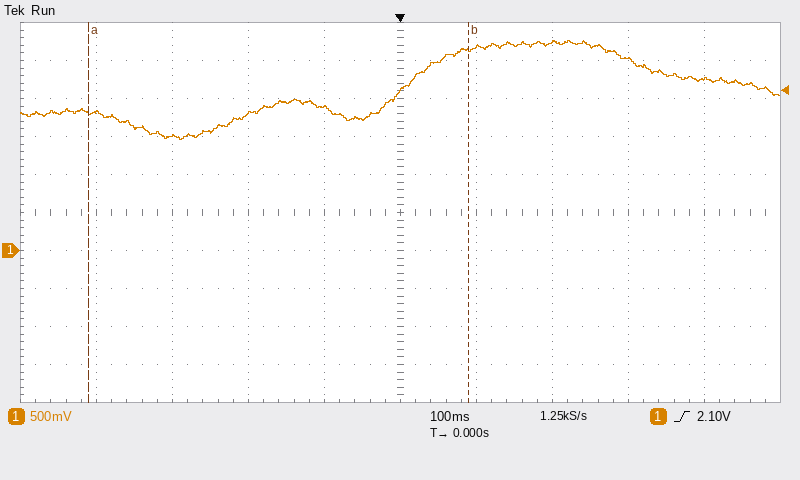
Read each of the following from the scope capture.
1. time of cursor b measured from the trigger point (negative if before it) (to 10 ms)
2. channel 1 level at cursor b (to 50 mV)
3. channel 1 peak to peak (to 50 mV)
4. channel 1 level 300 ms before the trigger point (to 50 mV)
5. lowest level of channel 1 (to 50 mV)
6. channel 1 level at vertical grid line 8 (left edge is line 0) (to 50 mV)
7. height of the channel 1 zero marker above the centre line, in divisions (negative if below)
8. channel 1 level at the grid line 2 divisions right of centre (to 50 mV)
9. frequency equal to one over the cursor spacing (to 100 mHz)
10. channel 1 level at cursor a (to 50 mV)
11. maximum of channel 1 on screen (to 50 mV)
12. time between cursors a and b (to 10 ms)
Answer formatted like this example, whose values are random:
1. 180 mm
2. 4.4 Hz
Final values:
1. +90 ms
2. 2.65 V
3. 1.30 V
4. 1.50 V
5. 1.45 V
6. 2.50 V
7. -1.0 div
8. 2.75 V
9. 2.0 Hz
10. 1.80 V
11. 2.75 V
12. 500 ms
